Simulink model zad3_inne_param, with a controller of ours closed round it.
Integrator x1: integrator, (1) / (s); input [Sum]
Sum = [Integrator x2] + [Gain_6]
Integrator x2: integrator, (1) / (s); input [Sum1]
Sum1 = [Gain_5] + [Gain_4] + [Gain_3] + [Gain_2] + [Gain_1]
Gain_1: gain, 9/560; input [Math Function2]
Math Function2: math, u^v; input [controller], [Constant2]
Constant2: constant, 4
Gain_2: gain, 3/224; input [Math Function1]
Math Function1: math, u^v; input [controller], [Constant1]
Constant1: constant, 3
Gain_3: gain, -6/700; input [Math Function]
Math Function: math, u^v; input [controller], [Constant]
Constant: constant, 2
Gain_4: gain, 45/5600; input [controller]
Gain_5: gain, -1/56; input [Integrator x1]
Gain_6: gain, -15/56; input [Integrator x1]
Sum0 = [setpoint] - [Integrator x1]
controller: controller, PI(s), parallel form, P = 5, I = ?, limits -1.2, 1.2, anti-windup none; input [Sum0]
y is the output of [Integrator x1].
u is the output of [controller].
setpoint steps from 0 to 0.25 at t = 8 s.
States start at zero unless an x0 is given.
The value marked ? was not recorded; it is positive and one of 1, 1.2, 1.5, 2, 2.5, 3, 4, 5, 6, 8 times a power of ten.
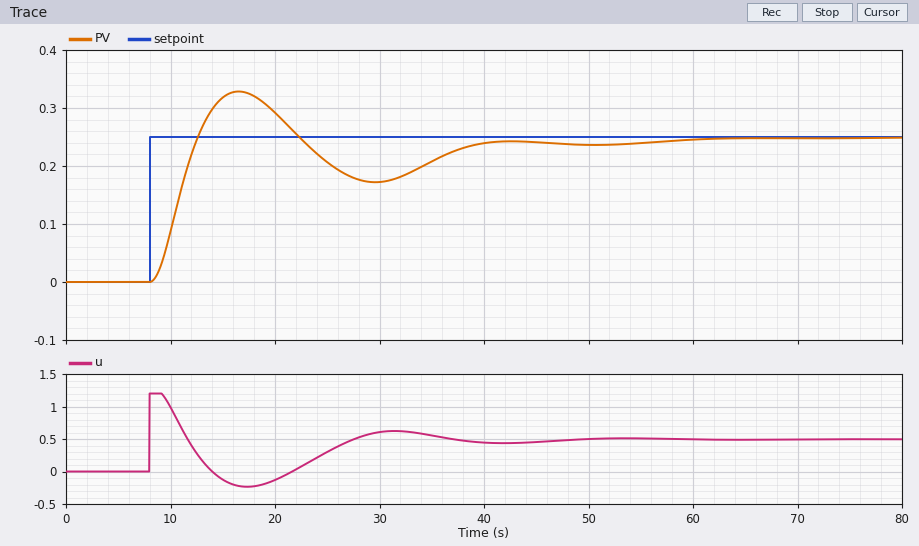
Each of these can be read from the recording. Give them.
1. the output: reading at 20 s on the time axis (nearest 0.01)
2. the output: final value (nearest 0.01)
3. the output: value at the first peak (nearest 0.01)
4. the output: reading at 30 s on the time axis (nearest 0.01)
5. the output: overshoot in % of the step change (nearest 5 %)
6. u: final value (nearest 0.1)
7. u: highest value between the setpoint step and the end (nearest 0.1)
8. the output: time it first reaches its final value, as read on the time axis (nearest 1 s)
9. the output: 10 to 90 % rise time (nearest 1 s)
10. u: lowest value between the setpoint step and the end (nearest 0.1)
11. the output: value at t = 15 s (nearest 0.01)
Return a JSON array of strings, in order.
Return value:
["0.29", "0.25", "0.33", "0.17", "30 %", "0.5", "1.2", "13 s", "3 s", "-0.2", "0.32"]
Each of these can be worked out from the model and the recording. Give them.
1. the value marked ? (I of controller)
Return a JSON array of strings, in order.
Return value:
["0.4"]
